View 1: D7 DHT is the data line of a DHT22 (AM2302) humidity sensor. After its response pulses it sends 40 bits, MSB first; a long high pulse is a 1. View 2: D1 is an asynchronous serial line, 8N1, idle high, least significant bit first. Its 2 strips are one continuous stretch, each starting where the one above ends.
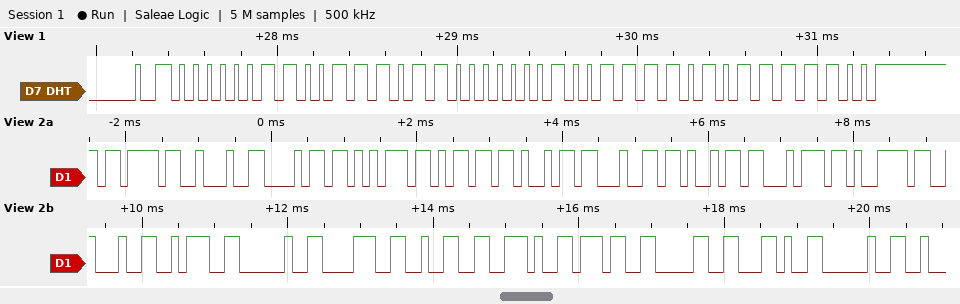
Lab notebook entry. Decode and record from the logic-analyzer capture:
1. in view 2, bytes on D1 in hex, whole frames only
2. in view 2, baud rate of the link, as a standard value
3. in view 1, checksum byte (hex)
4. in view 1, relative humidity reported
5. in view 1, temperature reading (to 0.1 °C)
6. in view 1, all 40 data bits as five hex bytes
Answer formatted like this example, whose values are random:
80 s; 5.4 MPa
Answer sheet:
7B 22 68 75 6D 69 64 69 74 79 22 3A 20 38 32 2E 37 30 2C 20; 9600 baud; 0x7C; 82.7 %; 31.7 °C; 03 3B 01 3D 7C
